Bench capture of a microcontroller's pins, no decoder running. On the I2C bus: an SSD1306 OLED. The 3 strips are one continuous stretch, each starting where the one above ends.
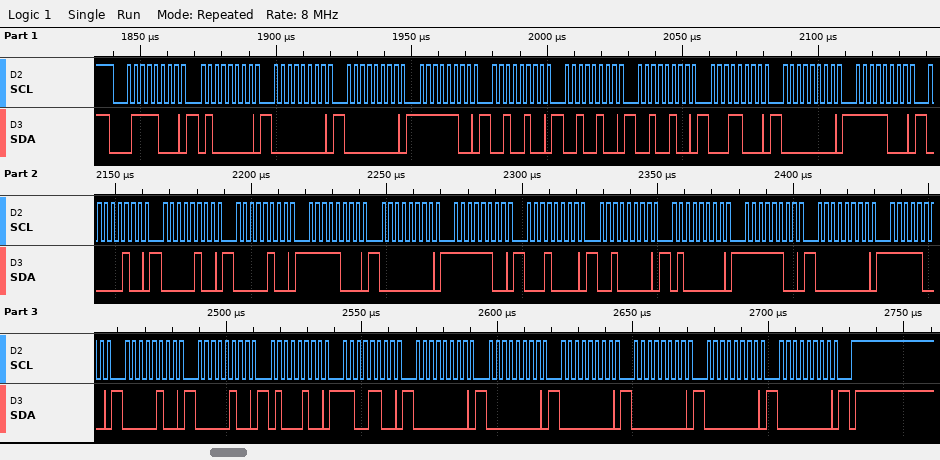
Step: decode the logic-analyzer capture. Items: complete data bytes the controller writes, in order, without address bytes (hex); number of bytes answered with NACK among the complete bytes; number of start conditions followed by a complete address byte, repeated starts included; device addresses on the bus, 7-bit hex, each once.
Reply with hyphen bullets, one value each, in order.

- 40 00 00 FC 24 24 24 18 00 F8 04 04 04 F8 00 FC 10 20 40 FC 00 F8 04 04 44 CC 00 00 00 00 00 00
- 0
- 1
- 0x3C
